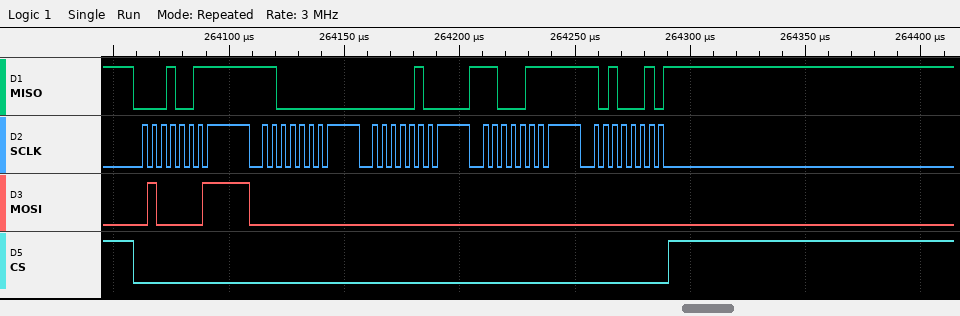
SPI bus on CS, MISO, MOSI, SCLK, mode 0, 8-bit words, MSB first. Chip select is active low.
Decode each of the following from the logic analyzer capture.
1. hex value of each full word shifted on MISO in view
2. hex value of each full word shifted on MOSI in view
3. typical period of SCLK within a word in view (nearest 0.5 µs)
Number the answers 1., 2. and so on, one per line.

1. 13, C0, 04, C7, A2
2. 41, 00, 00, 00, 00
3. 4 µs
